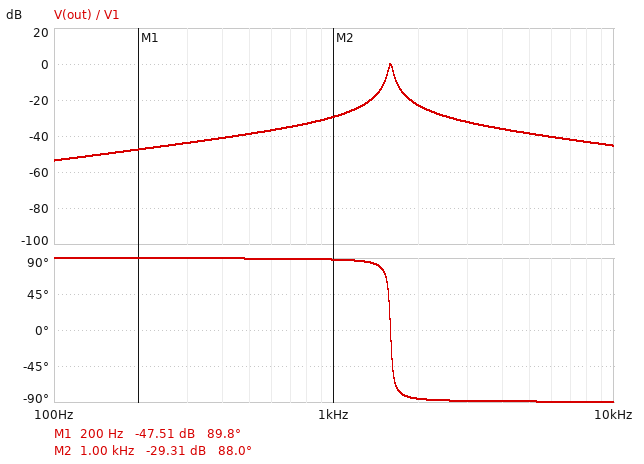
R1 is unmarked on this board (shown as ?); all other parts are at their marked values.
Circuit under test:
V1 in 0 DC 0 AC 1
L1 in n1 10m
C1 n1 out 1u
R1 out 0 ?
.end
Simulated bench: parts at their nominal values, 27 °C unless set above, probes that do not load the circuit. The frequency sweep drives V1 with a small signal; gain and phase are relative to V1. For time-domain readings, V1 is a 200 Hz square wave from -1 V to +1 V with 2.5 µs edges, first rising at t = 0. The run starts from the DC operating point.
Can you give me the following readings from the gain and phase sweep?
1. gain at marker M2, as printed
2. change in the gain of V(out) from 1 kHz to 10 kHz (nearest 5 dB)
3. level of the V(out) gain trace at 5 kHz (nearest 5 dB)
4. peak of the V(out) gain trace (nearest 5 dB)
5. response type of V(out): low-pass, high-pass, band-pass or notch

-29.31 dB
-15 dB
-40 dB
0 dB
band-pass
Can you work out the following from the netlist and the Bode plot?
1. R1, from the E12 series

3.3 Ω
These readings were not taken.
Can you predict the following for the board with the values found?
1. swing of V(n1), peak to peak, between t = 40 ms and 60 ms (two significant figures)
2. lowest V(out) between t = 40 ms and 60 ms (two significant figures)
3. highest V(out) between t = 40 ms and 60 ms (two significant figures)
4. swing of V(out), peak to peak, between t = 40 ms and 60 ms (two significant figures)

4.3 V
-39 mV
39 mV
78 mV
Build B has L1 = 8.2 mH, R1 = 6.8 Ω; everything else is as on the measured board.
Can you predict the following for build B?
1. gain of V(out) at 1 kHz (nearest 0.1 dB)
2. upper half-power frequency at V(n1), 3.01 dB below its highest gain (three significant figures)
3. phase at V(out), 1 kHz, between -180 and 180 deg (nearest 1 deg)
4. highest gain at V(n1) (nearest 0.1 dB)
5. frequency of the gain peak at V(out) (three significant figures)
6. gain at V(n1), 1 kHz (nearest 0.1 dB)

-24.0 dB
1.82 kHz
86 deg
22.5 dB
1.76 kHz
3.4 dB
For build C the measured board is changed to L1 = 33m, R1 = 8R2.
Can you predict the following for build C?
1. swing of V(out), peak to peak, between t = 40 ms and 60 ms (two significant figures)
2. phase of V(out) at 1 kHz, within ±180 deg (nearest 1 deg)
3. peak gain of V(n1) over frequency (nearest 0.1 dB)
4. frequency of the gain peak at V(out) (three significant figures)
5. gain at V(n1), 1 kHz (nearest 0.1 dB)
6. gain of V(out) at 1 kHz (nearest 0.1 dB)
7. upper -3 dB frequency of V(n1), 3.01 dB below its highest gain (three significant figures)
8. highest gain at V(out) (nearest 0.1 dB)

120 mV
-80 deg
26.9 dB
876 Hz
10.3 dB
-15.5 dB
895 Hz
0 dB
